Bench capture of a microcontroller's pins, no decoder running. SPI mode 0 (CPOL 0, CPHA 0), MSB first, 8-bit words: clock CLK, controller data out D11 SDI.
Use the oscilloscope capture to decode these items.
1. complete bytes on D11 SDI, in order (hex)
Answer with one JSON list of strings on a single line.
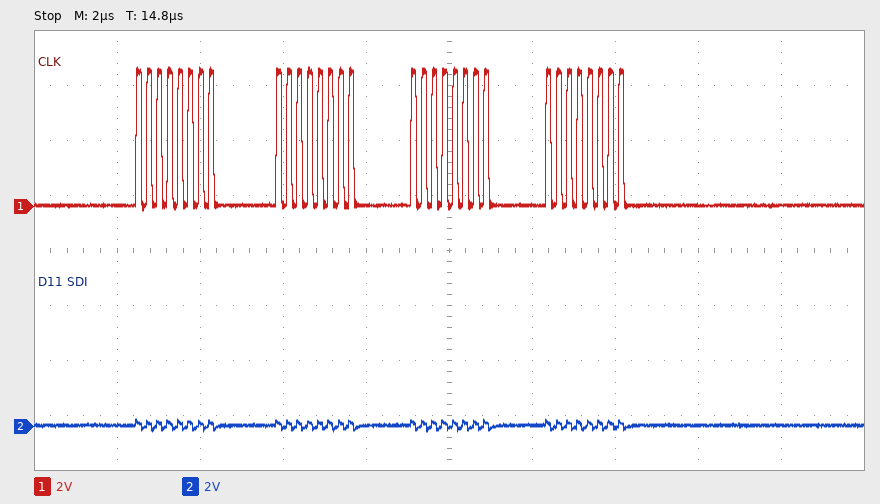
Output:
["00 00 00 00"]
